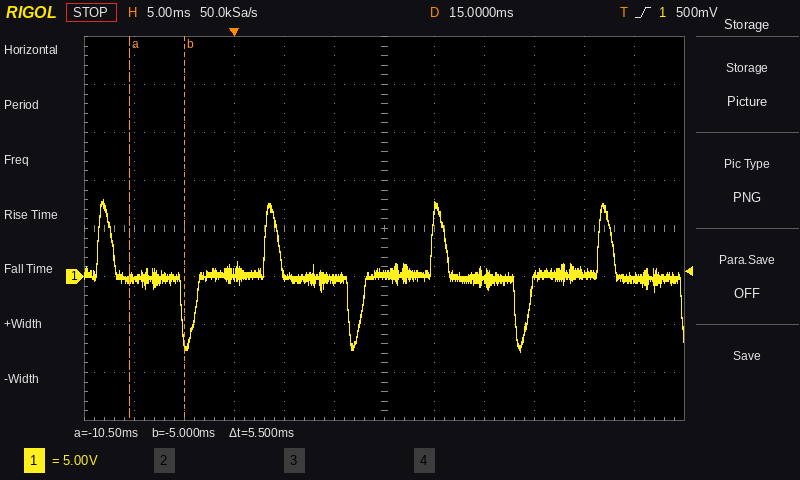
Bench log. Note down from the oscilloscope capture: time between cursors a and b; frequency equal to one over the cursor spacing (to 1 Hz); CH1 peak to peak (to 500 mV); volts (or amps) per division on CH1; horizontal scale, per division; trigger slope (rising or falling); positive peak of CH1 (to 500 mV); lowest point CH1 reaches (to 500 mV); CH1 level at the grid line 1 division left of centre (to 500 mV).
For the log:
5.5 ms
182 Hz
16.0 V
5 V
5 ms
rising
8.0 V
-8.0 V
-500 mV
